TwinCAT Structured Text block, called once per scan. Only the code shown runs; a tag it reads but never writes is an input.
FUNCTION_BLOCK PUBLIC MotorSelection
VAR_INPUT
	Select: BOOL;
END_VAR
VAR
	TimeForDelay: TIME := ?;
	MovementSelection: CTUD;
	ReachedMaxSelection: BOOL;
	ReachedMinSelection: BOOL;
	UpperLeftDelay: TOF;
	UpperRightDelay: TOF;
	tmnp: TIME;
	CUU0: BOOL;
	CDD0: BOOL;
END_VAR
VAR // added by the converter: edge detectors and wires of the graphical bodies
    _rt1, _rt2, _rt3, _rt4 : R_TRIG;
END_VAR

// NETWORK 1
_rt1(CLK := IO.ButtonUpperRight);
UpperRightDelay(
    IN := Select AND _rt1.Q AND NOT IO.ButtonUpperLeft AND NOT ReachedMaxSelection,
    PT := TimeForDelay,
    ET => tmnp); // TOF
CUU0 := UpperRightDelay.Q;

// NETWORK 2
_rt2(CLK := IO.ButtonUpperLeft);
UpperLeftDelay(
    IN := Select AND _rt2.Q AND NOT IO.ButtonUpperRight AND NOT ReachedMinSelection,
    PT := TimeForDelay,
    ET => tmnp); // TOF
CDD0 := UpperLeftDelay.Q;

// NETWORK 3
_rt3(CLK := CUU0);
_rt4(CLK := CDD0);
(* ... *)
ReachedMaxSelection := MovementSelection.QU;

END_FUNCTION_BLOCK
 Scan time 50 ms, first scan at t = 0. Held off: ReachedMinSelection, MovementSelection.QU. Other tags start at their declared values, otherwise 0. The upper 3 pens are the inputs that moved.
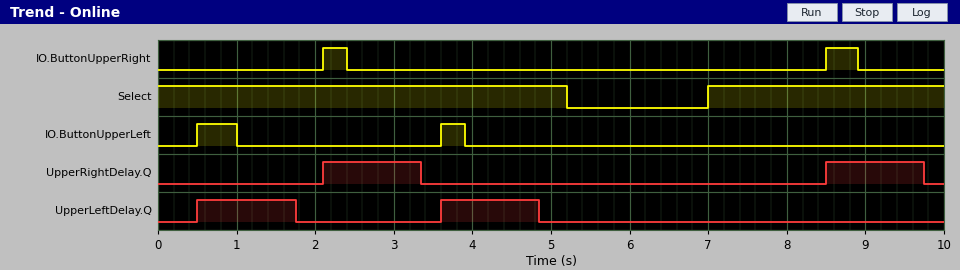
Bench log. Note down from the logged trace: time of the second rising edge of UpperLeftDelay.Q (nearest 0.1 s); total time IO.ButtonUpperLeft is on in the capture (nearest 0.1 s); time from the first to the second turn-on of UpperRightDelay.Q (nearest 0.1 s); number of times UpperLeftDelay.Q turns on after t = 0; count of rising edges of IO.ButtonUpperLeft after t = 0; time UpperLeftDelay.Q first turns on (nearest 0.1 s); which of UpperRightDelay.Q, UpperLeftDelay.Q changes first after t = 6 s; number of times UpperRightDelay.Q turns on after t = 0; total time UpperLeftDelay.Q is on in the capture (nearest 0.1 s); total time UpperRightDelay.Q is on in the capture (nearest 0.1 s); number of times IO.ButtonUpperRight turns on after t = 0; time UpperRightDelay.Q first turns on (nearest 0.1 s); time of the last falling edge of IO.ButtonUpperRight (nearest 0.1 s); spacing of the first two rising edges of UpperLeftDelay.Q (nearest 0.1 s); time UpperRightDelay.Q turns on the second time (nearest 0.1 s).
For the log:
3.6 s
0.8 s
6.4 s
2
2
0.5 s
UpperRightDelay.Q
2
2.5 s
2.5 s
2
2.1 s
8.9 s
3.1 s
8.5 s
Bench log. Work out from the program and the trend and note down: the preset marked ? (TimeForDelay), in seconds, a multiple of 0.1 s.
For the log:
1.2 s
